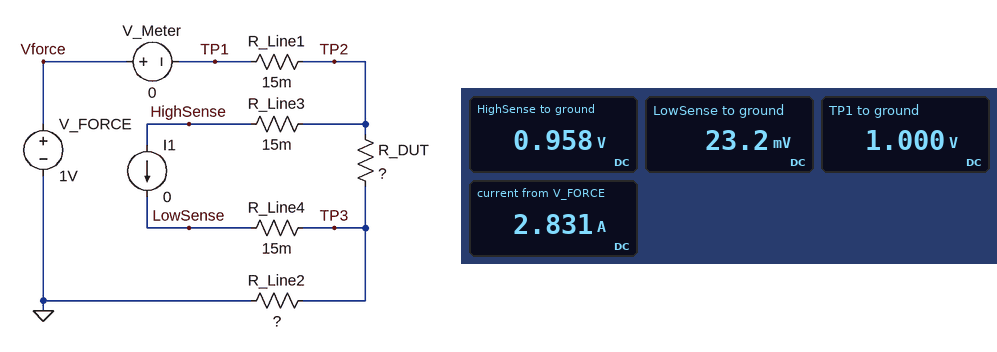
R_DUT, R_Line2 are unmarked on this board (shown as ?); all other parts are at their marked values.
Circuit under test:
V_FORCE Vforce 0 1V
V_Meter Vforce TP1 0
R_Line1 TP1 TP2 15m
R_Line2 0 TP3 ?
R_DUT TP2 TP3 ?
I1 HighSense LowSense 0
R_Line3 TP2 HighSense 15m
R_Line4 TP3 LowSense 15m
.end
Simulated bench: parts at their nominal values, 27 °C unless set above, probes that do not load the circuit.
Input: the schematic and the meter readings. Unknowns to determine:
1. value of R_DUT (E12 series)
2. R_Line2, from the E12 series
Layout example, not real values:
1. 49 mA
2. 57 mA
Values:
1. 0.33 Ω
2. 8.2 mΩ
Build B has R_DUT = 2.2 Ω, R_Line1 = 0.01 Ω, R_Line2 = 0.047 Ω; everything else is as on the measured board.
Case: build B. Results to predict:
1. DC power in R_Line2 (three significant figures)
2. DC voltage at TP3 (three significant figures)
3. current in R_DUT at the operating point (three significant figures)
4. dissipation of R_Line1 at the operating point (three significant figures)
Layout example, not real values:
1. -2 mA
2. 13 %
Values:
1. 9.23 mW
2. 20.8 mV
3. 443 mA
4. 1.96 mW
